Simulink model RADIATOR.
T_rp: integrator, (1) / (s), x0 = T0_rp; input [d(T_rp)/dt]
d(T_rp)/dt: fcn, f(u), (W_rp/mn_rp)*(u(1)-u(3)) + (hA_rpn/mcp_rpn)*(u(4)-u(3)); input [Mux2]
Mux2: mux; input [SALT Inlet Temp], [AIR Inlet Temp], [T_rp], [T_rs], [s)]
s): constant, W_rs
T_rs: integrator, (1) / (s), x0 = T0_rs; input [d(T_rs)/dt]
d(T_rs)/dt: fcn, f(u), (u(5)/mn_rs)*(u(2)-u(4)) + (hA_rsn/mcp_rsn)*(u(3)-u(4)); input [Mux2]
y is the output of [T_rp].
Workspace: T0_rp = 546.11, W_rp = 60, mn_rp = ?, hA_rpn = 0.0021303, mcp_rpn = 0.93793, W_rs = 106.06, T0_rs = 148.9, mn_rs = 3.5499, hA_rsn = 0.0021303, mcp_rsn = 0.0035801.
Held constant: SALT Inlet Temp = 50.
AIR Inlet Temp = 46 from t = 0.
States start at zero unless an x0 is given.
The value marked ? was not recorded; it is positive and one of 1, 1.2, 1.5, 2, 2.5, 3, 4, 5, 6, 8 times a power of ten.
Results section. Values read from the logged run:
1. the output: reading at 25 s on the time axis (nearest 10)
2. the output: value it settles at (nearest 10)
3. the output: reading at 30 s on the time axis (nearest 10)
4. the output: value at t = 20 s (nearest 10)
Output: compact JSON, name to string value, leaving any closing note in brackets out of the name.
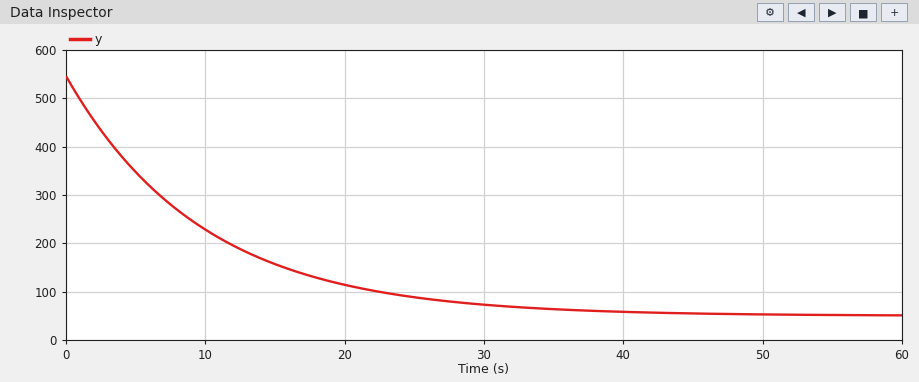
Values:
{"the output: reading at 25 s on the time axis": "90", "the output: value it settles at": "50", "the output: reading at 30 s on the time axis": "70", "the output: value at t = 20 s": "110"}
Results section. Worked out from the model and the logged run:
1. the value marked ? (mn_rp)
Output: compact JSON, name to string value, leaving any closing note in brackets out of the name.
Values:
{"the value marked ?": "600"}
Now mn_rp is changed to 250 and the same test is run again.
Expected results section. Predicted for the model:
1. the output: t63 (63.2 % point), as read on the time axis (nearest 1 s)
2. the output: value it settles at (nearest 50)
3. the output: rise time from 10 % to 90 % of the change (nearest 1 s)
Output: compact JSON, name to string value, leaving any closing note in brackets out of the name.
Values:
{"the output: t63 (63.2 % point), as read on the time axis": "4 s", "the output: value it settles at": "50", "the output: rise time from 10 % to 90 % of the change": "9 s"}
